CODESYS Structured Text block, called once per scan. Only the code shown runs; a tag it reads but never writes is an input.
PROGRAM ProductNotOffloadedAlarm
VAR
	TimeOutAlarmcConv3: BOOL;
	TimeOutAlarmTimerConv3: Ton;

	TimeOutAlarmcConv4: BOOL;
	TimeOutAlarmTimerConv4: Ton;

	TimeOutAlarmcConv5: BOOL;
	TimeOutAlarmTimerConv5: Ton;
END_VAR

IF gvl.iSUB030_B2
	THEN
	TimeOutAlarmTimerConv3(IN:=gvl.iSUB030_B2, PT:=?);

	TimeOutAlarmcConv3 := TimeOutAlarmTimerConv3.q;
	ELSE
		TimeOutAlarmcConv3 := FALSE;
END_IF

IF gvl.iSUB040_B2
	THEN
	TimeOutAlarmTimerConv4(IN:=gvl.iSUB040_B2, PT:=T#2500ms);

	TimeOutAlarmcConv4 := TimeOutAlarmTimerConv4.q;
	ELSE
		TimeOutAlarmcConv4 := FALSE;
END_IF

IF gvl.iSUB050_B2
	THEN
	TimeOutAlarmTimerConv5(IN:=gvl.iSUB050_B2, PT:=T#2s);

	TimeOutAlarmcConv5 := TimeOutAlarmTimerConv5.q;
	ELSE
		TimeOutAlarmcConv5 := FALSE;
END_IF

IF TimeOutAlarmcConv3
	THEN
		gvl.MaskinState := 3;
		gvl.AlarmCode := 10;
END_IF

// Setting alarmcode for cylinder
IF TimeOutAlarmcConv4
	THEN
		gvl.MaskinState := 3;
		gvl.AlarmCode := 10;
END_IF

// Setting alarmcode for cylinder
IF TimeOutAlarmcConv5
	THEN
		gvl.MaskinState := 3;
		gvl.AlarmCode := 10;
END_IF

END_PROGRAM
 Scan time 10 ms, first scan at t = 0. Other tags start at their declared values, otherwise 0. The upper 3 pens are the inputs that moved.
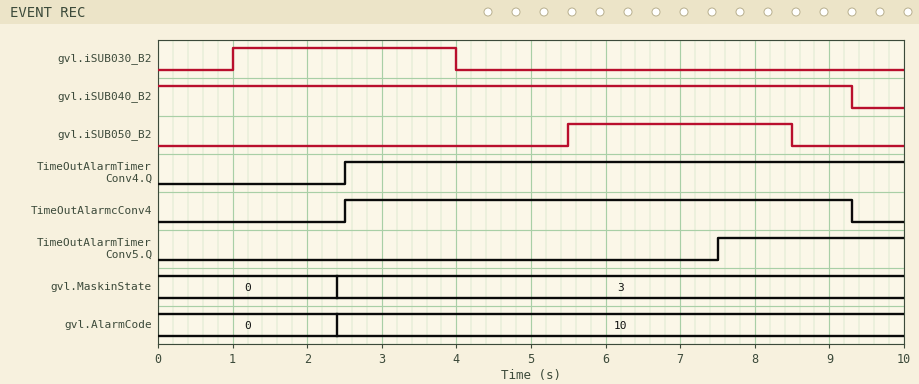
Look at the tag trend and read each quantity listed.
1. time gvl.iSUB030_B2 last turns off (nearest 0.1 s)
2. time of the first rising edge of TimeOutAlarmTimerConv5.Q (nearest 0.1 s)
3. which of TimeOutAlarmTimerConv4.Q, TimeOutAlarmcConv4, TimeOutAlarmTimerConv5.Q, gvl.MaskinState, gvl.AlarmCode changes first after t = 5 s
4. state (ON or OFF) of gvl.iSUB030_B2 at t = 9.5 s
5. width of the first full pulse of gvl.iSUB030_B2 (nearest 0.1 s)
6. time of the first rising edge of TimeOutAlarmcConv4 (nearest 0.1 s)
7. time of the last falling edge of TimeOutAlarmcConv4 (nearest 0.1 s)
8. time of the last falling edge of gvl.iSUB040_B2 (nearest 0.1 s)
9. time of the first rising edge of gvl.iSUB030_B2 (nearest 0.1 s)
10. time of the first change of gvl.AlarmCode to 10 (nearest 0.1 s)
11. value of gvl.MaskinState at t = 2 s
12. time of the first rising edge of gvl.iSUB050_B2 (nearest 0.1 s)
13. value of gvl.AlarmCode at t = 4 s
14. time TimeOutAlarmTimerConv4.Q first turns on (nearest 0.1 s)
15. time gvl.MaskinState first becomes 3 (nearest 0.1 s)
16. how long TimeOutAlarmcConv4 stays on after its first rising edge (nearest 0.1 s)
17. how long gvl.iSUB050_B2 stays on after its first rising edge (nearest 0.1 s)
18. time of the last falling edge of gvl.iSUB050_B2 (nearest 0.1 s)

4.0 s
7.5 s
TimeOutAlarmTimerConv5.Q
OFF
3.0 s
2.5 s
9.3 s
9.3 s
1.0 s
2.4 s
0
5.5 s
10
2.5 s
2.4 s
6.8 s
3.0 s
8.5 s
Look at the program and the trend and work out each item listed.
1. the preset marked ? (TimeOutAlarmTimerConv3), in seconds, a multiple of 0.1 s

1.4 s
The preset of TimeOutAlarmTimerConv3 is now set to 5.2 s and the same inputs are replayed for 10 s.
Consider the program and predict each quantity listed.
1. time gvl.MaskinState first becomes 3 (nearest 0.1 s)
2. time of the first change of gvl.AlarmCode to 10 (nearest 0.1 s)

2.5 s
2.5 s
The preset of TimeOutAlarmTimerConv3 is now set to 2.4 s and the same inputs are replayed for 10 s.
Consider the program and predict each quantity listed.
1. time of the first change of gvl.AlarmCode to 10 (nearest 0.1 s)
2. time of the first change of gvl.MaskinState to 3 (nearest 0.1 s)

2.5 s
2.5 s
